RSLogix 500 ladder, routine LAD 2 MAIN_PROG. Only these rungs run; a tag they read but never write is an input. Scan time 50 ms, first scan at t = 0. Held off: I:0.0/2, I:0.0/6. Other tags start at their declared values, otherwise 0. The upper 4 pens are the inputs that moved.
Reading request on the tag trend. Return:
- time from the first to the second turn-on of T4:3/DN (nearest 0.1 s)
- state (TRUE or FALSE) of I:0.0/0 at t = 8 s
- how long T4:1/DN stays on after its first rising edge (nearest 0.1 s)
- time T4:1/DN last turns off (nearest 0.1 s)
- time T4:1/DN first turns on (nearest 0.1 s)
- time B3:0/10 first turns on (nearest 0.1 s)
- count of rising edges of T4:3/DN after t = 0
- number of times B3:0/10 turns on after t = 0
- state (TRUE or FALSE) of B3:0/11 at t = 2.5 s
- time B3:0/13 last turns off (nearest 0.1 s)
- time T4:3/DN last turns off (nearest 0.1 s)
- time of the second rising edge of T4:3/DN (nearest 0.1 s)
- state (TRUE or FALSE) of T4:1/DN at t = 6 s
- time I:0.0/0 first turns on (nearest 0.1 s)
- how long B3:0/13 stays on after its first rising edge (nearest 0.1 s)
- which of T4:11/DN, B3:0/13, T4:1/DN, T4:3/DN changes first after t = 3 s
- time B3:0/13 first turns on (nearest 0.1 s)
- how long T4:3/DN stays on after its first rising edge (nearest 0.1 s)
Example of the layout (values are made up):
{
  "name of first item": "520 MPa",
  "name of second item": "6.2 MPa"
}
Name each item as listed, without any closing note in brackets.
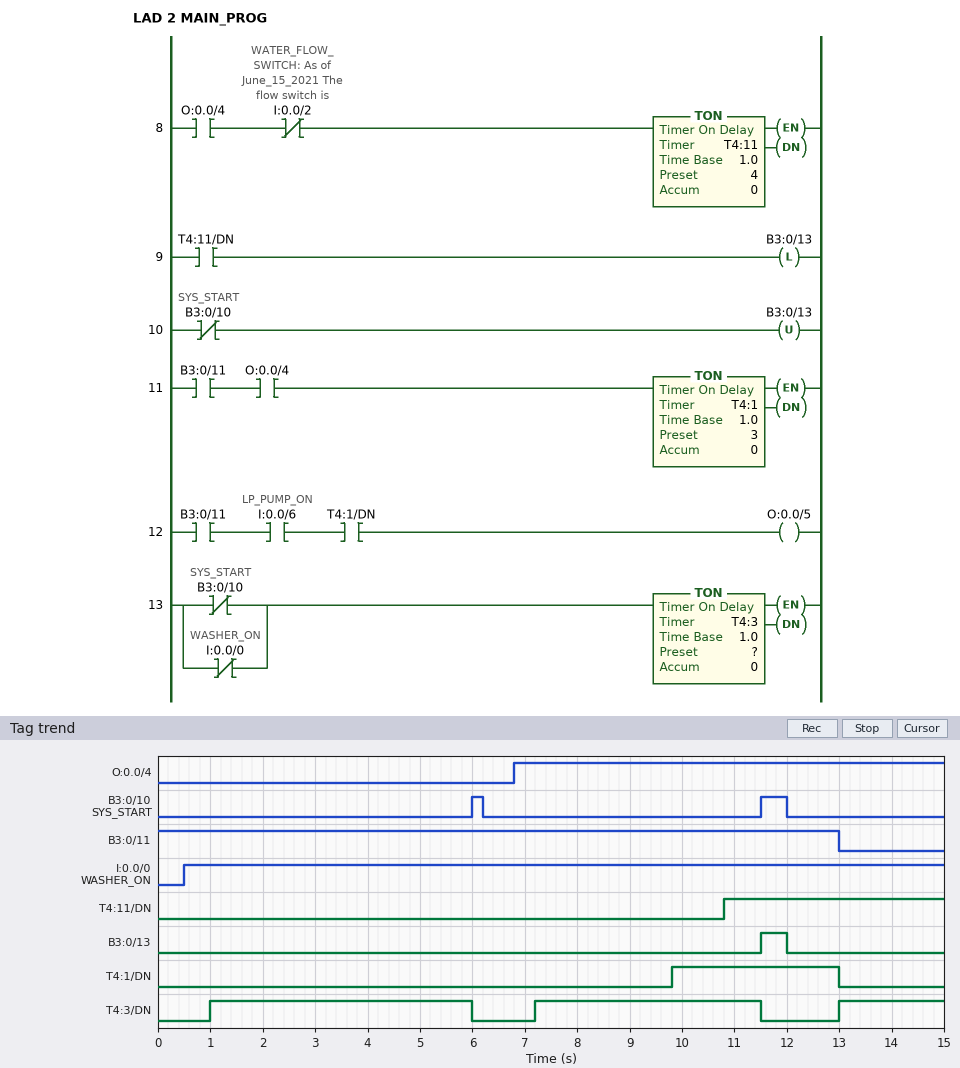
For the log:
{
  "time from the first to the second turn-on of T4:3/DN": "6.2 s",
  "state (TRUE or FALSE) of I:0.0/0 at t = 8 s": "TRUE",
  "how long T4:1/DN stays on after its first rising edge": "3.2 s",
  "time T4:1/DN last turns off": "13.0 s",
  "time T4:1/DN first turns on": "9.8 s",
  "time B3:0/10 first turns on": "6.0 s",
  "count of rising edges of T4:3/DN after t = 0": "3",
  "number of times B3:0/10 turns on after t = 0": "2",
  "state (TRUE or FALSE) of B3:0/11 at t = 2.5 s": "TRUE",
  "time B3:0/13 last turns off": "12.0 s",
  "time T4:3/DN last turns off": "11.5 s",
  "time of the second rising edge of T4:3/DN": "7.2 s",
  "state (TRUE or FALSE) of T4:1/DN at t = 6 s": "FALSE",
  "time I:0.0/0 first turns on": "0.5 s",
  "how long B3:0/13 stays on after its first rising edge": "0.5 s",
  "which of T4:11/DN, B3:0/13, T4:1/DN, T4:3/DN changes first after t = 3 s": "T4:3/DN",
  "time B3:0/13 first turns on": "11.5 s",
  "how long T4:3/DN stays on after its first rising edge": "5.0 s"
}
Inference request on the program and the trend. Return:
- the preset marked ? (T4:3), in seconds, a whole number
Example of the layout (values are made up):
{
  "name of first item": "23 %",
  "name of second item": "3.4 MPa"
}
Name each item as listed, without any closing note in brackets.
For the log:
{
  "the preset marked ? (T4:3), in seconds, a whole number": "1 s"
}
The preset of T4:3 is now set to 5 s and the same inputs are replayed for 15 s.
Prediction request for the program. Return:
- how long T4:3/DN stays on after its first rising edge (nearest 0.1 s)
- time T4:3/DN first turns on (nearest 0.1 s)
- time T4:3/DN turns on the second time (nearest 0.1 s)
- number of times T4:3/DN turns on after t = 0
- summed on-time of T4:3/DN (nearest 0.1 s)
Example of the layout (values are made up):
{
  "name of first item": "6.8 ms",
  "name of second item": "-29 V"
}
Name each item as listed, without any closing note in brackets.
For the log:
{
  "how long T4:3/DN stays on after its first rising edge": "1.0 s",
  "time T4:3/DN first turns on": "5.0 s",
  "time T4:3/DN turns on the second time": "11.2 s",
  "number of times T4:3/DN turns on after t = 0": "2",
  "summed on-time of T4:3/DN": "1.3 s"
}
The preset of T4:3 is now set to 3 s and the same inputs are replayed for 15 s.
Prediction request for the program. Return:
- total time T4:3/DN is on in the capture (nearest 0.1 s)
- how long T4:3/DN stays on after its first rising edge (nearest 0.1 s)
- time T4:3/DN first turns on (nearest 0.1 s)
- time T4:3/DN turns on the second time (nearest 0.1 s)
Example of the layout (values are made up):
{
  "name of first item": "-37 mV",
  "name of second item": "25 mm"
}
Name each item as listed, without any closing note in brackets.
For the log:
{
  "total time T4:3/DN is on in the capture": "5.3 s",
  "how long T4:3/DN stays on after its first rising edge": "3.0 s",
  "time T4:3/DN first turns on": "3.0 s",
  "time T4:3/DN turns on the second time": "9.2 s"
}
